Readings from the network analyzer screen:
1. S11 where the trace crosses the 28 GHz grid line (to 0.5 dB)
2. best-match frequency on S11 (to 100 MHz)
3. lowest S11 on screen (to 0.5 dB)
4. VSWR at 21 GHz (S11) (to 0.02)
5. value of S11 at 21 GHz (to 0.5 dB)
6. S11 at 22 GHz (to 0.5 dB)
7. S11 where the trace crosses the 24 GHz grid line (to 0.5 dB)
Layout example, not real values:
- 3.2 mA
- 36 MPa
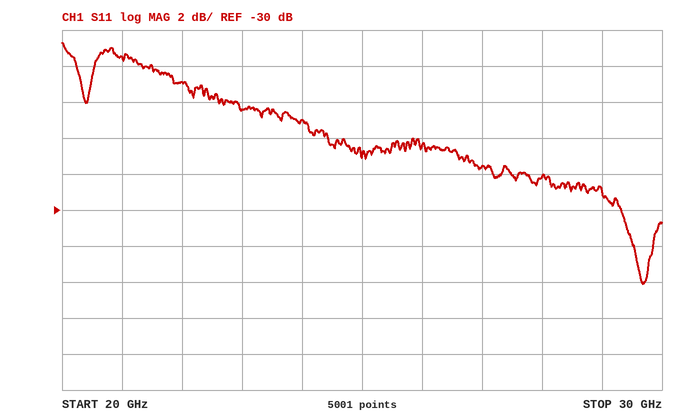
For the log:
- -28.0 dB
- 29.7 GHz
- -34.0 dB
- 1.18
- -21.5 dB
- -23.0 dB
- -25.0 dB
